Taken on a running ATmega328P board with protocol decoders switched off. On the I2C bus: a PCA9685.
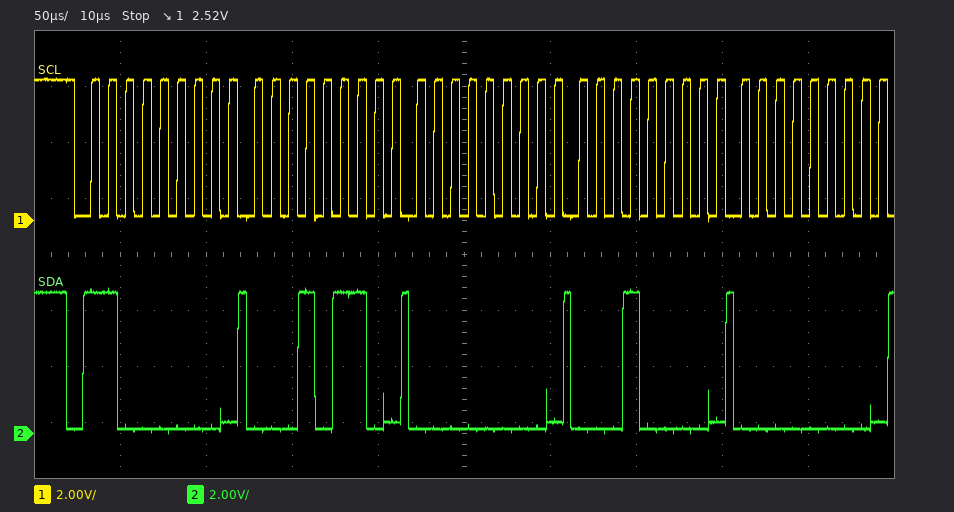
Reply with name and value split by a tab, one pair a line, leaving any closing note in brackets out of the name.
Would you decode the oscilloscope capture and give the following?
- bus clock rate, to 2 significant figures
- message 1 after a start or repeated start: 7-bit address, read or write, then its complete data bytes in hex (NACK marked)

bus clock rate, to 2 significant figures	100 kHz
message 1 after a start or repeated start: 7-bit address, read or write, then its complete data bytes in hex	0x60 write: 16 00 10 00
